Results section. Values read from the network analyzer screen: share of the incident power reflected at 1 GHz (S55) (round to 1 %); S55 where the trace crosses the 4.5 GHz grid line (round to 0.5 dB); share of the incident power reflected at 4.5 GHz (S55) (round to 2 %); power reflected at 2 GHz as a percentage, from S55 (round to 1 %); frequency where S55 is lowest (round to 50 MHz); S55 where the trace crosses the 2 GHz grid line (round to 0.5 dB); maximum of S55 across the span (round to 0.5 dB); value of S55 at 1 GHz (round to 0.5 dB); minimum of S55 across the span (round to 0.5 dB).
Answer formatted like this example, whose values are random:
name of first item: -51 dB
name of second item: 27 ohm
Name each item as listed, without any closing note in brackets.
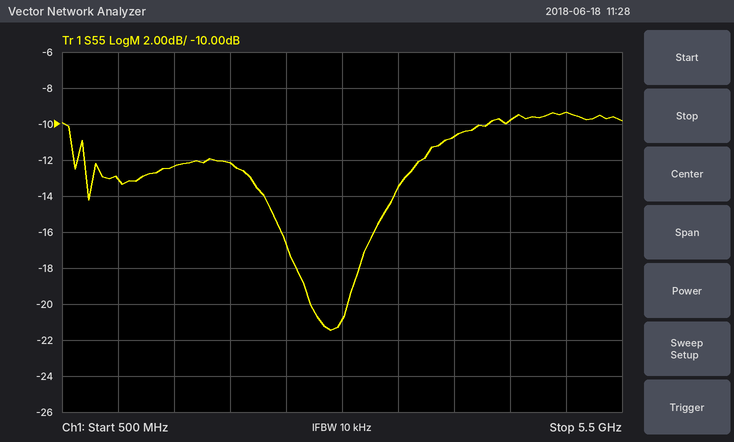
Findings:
share of the incident power reflected at 1 GHz (S55): 5 %
S55 where the trace crosses the 4.5 GHz grid line: -10.0 dB
share of the incident power reflected at 4.5 GHz (S55): 10 %
power reflected at 2 GHz as a percentage, from S55: 6 %
frequency where S55 is lowest: 2.90 GHz
S55 where the trace crosses the 2 GHz grid line: -12.0 dB
maximum of S55 across the span: -9.5 dB
value of S55 at 1 GHz: -13.0 dB
minimum of S55 across the span: -21.5 dB
